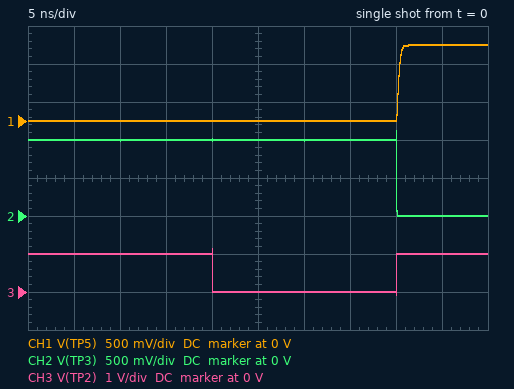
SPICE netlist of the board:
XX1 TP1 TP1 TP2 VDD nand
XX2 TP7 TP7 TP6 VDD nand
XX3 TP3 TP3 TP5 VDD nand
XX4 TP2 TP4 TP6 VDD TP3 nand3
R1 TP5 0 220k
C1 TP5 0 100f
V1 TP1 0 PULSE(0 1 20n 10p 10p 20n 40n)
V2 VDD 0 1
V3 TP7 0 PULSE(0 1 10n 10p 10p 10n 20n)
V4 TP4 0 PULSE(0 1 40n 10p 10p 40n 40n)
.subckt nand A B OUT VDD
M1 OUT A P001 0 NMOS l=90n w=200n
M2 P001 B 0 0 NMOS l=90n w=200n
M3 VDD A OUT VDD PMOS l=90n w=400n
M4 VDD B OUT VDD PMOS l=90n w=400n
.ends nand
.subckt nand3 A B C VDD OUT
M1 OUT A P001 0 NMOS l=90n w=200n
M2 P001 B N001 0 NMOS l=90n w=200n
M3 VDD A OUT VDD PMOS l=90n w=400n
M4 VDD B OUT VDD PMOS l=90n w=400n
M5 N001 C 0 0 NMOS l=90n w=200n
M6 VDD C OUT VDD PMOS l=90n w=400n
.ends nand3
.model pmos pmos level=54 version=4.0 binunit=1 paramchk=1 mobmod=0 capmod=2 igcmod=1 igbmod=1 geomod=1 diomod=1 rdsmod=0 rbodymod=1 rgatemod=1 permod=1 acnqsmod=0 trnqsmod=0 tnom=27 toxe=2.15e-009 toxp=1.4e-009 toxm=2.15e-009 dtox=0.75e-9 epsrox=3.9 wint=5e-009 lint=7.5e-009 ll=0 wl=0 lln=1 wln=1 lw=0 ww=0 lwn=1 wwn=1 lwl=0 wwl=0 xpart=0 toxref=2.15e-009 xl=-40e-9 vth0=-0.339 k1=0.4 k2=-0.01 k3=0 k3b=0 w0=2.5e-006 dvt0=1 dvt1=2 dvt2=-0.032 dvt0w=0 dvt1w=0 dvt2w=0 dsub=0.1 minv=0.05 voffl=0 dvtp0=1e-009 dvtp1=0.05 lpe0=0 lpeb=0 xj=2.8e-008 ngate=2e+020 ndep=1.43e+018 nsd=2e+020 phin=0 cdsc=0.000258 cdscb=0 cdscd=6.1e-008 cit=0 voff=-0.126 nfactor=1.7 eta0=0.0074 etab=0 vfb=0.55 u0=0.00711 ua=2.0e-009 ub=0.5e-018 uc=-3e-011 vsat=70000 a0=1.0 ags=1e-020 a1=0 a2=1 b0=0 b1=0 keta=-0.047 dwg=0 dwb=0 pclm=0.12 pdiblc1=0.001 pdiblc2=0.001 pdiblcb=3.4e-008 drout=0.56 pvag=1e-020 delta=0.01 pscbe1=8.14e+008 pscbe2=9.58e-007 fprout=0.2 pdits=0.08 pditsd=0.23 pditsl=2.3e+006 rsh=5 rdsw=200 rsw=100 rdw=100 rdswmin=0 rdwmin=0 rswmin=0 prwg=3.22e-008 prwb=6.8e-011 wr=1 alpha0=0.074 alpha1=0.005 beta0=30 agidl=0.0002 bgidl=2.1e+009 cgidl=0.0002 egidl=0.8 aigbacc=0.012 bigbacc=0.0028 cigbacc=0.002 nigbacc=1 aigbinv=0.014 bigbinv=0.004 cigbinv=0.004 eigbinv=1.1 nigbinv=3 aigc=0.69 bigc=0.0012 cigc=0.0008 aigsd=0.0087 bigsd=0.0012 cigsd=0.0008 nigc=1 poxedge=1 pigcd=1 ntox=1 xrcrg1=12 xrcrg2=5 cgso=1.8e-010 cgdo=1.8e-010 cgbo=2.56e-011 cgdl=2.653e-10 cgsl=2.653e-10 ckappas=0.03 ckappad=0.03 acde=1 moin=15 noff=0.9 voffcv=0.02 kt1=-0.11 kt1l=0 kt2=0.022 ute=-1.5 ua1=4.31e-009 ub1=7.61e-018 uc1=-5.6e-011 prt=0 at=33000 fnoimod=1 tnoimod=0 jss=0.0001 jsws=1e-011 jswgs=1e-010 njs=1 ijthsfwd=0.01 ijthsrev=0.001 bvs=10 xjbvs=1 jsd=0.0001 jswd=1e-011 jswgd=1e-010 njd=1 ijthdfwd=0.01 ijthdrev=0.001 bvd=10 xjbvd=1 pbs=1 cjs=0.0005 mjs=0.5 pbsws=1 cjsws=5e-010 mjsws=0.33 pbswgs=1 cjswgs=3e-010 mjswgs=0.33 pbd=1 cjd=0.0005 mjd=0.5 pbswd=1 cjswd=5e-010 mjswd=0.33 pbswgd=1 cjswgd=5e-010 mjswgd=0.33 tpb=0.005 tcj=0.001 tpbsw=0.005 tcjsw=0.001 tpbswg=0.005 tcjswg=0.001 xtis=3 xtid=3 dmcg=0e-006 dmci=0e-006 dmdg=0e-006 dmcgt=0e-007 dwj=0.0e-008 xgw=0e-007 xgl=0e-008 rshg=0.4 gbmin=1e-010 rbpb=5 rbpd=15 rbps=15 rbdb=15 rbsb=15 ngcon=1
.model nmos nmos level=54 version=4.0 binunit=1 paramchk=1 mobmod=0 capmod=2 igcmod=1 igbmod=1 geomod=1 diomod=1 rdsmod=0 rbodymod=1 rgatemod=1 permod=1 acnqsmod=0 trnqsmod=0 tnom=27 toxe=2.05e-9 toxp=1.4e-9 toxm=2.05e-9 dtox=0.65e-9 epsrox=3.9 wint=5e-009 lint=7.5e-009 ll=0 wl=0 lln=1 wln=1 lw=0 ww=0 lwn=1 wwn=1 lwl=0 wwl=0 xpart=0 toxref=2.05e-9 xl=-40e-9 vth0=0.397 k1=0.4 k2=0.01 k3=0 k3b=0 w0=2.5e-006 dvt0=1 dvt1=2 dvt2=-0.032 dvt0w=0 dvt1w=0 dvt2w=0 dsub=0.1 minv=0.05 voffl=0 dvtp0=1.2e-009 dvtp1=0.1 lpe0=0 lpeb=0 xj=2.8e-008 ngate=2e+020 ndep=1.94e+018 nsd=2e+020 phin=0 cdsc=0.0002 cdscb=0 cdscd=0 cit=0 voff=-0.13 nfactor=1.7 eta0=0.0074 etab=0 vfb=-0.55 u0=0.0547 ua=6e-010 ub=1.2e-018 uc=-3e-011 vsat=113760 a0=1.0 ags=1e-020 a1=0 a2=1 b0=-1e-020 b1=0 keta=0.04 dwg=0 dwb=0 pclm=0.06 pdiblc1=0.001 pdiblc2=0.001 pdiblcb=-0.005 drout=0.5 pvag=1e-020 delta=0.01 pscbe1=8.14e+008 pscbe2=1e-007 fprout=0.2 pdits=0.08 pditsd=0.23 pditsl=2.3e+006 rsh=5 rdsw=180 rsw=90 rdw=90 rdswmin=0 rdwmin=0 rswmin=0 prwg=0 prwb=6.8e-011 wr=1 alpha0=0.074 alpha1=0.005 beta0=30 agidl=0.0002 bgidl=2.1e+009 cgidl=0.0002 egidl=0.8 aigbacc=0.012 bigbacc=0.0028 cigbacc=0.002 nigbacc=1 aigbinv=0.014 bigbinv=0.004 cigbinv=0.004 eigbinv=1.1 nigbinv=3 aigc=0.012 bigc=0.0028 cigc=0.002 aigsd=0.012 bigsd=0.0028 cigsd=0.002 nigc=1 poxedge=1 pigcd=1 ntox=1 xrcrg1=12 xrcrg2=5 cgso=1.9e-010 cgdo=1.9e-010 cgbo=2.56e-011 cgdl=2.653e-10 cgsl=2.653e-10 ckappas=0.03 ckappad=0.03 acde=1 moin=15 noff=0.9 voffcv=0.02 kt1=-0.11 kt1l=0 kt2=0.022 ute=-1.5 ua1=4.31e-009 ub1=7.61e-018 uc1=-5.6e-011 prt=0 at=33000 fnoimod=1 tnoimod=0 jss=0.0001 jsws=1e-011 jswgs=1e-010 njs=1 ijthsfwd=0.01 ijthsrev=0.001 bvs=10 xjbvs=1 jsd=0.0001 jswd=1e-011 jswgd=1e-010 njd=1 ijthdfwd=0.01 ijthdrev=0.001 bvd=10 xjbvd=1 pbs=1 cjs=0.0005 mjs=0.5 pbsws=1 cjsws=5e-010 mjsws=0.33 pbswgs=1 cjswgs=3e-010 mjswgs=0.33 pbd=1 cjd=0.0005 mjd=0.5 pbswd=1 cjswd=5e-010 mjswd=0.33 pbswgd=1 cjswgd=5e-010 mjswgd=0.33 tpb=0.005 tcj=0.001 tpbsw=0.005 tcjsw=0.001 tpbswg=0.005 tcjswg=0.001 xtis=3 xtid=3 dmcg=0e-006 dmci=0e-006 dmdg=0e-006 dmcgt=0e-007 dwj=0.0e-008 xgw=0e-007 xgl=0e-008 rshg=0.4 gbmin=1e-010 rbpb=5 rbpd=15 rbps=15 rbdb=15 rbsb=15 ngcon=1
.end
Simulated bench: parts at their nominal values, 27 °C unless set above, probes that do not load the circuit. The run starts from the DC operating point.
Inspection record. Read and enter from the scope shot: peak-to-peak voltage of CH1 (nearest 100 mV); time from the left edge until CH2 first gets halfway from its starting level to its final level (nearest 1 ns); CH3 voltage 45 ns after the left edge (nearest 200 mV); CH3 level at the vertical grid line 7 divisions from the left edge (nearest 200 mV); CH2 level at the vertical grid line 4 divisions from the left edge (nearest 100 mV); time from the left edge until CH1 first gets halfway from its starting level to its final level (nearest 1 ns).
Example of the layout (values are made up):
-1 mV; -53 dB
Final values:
1.0 V; 40 ns; 1.0 V; 0 V; 1.0 V; 40 ns
